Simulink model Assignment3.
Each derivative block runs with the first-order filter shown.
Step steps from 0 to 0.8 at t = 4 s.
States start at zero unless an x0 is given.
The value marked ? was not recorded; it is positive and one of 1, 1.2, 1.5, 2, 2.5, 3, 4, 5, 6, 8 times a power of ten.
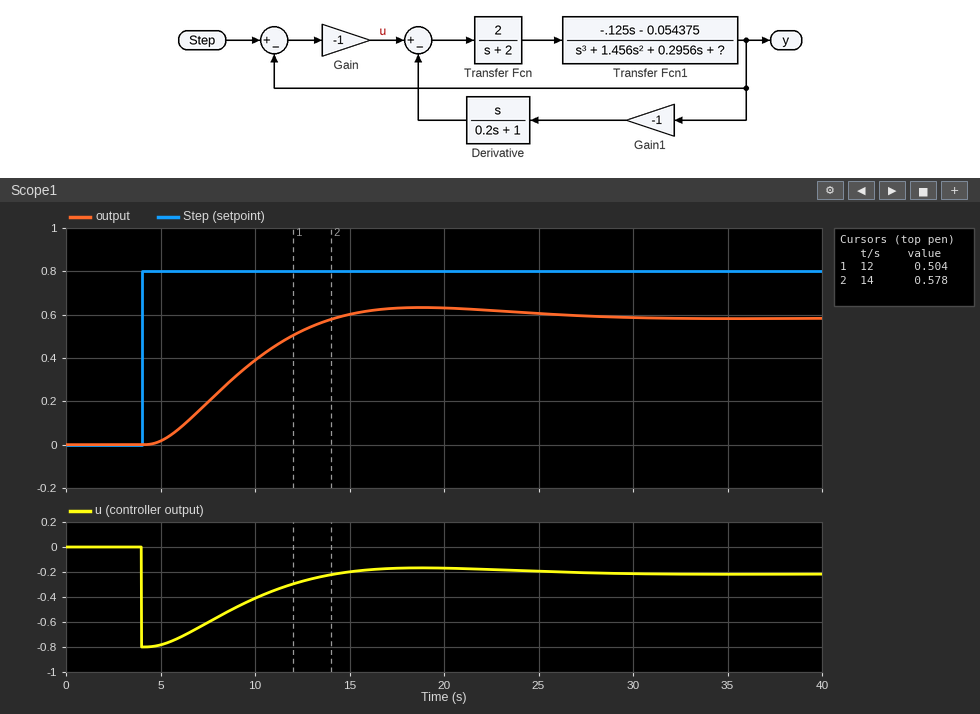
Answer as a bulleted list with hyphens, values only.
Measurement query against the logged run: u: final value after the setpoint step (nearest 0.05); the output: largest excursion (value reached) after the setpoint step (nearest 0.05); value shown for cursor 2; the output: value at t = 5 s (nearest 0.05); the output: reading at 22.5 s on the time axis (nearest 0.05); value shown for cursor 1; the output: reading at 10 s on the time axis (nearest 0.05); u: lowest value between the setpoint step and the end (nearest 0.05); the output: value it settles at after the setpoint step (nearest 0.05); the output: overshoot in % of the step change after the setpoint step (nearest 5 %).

- -0.20
- 0.65
- 0.578
- 0.00
- 0.60
- 0.504
- 0.40
- -0.80
- 0.60
- 10 %
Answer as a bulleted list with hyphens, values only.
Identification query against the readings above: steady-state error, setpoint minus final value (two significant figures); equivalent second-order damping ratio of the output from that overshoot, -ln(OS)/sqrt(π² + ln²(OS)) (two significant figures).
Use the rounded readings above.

- 0.20
- 0.59
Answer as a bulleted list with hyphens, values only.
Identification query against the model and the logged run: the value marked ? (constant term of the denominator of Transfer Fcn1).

- 0.02
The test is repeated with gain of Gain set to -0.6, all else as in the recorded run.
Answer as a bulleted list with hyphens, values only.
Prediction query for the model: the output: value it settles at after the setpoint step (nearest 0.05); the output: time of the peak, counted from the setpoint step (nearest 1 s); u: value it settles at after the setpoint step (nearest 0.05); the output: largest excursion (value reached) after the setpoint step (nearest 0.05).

- 0.50
- 20 s
- -0.20
- 0.50
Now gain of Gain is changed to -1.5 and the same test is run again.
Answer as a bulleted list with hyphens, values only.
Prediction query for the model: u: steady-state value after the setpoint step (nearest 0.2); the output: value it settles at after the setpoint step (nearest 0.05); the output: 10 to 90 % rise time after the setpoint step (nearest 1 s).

- -0.2
- 0.65
- 5 s
